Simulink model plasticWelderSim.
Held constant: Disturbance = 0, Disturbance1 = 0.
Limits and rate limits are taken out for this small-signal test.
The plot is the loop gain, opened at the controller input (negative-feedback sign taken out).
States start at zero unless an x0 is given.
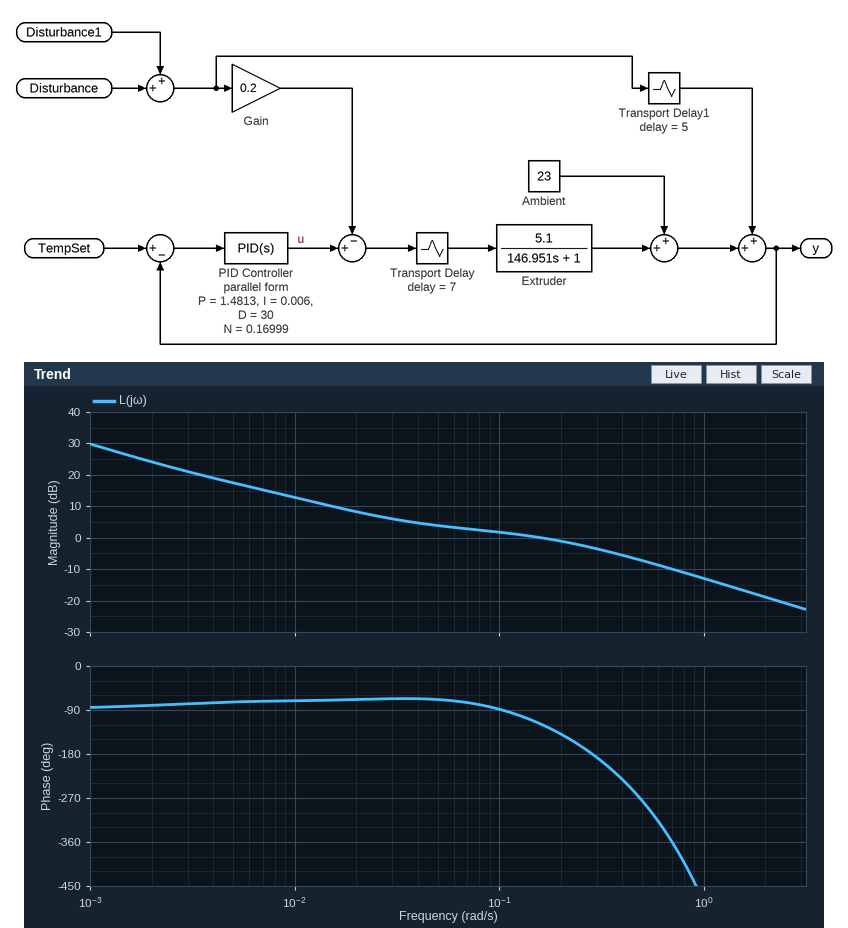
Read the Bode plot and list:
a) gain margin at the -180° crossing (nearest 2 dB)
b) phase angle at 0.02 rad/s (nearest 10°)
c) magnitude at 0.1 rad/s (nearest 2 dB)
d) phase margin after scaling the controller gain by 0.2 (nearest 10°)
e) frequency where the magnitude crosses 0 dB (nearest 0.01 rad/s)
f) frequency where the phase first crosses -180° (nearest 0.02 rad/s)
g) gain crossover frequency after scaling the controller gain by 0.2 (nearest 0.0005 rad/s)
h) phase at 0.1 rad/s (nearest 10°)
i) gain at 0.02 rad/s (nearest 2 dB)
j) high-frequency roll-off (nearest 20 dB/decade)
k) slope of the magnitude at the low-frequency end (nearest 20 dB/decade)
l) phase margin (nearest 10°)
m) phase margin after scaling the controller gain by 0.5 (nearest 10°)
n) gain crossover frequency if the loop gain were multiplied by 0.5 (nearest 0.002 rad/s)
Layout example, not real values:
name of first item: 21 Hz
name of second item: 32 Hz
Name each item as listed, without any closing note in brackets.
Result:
gain margin at the -180° crossing: 4 dB
phase angle at 0.02 rad/s: -70°
magnitude at 0.1 rad/s: 2 dB
phase margin after scaling the controller gain by 0.2: 110°
frequency where the magnitude crosses 0 dB: 0.16 rad/s
frequency where the phase first crosses -180°: 0.28 rad/s
gain crossover frequency after scaling the controller gain by 0.2: 0.0085 rad/s
phase at 0.1 rad/s: -90°
gain at 0.02 rad/s: 8 dB
high-frequency roll-off: -20 dB/decade
slope of the magnitude at the low-frequency end: -20 dB/decade
phase margin: 60°
phase margin after scaling the controller gain by 0.5: 110°
gain crossover frequency if the loop gain were multiplied by 0.5: 0.030 rad/s
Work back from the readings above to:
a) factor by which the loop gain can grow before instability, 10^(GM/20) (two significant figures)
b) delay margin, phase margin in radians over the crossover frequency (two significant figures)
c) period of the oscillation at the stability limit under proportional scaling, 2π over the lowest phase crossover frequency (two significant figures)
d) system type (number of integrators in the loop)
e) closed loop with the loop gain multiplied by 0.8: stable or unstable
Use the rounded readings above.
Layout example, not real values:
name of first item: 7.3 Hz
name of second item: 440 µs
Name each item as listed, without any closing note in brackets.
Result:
factor by which the loop gain can grow before instability, 10^(GM/20): 1.6
delay margin, phase margin in radians over the crossover frequency: 6.5 s
period of the oscillation at the stability limit under proportional scaling, 2π over the lowest phase crossover frequency: 22 s
system type: 1
closed loop with the loop gain multiplied by 0.8: stable or unstable: stable
